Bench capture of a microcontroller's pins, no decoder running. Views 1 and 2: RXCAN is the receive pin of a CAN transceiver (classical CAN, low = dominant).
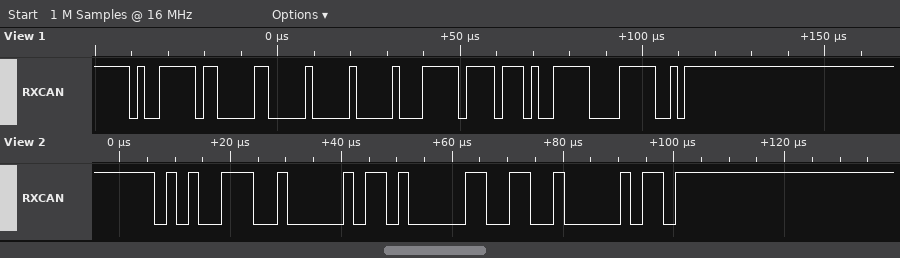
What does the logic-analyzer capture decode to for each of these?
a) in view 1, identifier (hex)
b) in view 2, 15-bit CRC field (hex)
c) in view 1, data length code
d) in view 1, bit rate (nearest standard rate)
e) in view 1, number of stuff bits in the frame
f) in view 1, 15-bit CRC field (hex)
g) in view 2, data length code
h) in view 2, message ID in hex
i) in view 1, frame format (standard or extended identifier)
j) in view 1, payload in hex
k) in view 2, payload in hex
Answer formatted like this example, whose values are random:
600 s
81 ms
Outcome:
0x4FE
0x4C81
4
500 kbit/s
8
0x3E3E
1
0x539
standard
00 00 FF BA
A0
